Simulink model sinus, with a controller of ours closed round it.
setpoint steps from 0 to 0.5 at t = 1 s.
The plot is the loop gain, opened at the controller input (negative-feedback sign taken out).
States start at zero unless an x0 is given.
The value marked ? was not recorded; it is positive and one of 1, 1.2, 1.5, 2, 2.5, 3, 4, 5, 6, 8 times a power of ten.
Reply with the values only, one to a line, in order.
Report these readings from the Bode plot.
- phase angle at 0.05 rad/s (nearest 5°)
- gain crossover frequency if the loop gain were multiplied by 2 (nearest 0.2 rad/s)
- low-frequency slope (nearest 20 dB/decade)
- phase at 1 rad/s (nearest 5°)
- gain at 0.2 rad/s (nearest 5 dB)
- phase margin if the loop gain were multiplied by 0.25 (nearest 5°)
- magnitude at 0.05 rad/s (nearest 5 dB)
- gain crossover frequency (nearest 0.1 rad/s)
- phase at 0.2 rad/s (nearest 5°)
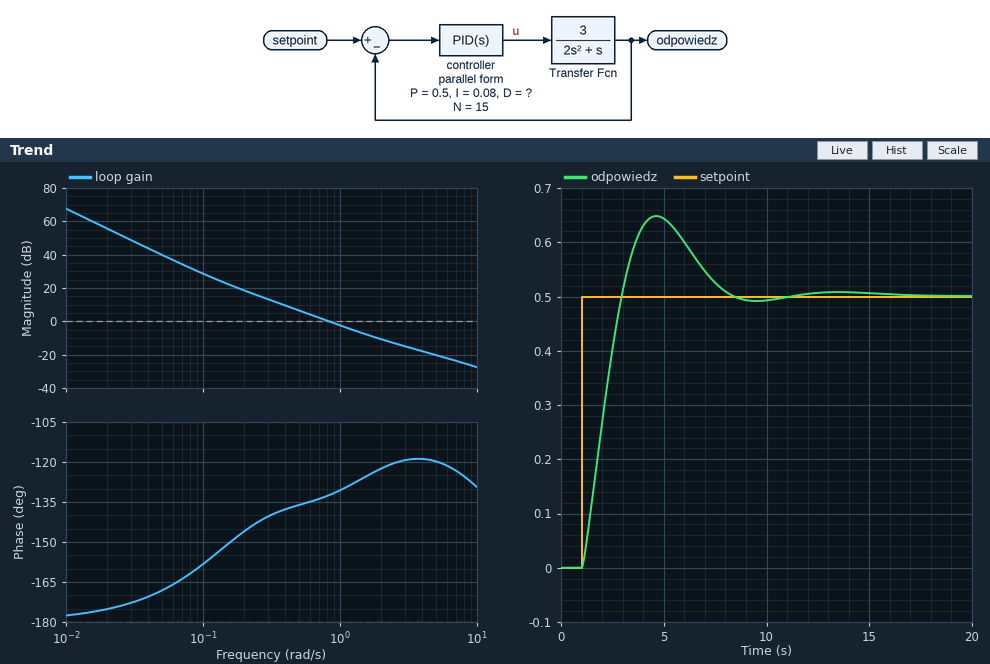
-170°
1.4 rad/s
-40 dB/decade
-130°
20 dB
40°
40 dB
0.8 rad/s
-145°
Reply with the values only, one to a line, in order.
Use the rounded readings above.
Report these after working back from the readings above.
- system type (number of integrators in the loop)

2
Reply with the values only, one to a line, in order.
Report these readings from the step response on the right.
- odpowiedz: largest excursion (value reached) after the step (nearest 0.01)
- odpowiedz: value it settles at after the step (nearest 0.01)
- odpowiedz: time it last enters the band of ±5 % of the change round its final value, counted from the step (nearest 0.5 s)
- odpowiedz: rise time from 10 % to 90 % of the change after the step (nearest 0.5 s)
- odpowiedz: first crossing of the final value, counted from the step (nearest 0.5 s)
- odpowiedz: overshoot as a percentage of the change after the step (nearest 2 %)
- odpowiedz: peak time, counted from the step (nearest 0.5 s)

0.65
0.50
6.5 s
1.5 s
2.0 s
30 %
3.5 s
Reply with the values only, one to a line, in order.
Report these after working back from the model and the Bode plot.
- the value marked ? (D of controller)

0.3
